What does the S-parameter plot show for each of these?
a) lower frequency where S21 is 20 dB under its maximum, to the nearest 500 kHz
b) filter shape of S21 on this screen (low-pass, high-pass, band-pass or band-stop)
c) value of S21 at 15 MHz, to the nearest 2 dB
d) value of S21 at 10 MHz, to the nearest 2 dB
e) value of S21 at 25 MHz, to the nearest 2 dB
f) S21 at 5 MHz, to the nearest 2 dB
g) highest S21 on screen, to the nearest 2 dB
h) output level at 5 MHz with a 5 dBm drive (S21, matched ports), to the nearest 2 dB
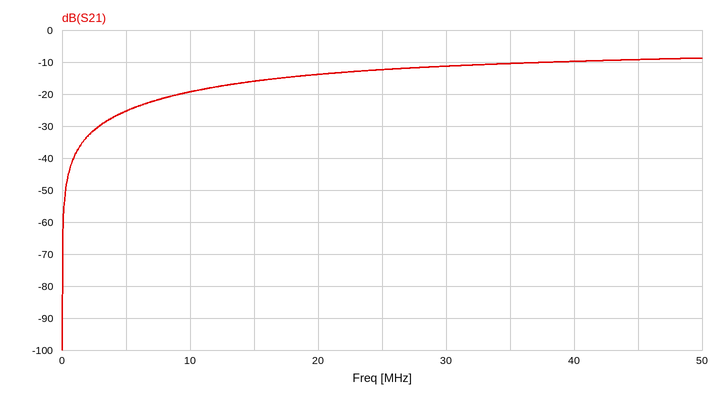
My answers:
3.5 MHz
high-pass
-16 dB
-20 dB
-12 dB
-26 dB
-8 dB
-20 dBm
